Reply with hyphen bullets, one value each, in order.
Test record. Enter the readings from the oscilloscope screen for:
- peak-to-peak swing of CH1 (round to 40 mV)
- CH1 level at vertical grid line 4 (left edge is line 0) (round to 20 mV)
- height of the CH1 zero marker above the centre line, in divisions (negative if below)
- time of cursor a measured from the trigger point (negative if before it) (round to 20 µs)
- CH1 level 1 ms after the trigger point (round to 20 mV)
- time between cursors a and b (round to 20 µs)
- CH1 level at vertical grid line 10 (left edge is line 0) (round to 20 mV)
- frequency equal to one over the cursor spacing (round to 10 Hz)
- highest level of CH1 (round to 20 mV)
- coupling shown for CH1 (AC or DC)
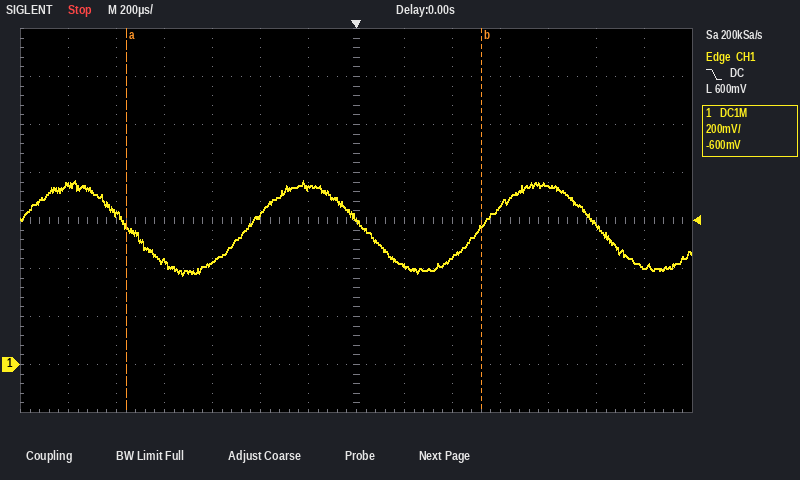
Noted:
- 400 mV
- 420 mV
- -3.0 div
- -960 µs
- 580 mV
- 1.48 ms
- 660 mV
- 680 Hz
- 760 mV
- DC
